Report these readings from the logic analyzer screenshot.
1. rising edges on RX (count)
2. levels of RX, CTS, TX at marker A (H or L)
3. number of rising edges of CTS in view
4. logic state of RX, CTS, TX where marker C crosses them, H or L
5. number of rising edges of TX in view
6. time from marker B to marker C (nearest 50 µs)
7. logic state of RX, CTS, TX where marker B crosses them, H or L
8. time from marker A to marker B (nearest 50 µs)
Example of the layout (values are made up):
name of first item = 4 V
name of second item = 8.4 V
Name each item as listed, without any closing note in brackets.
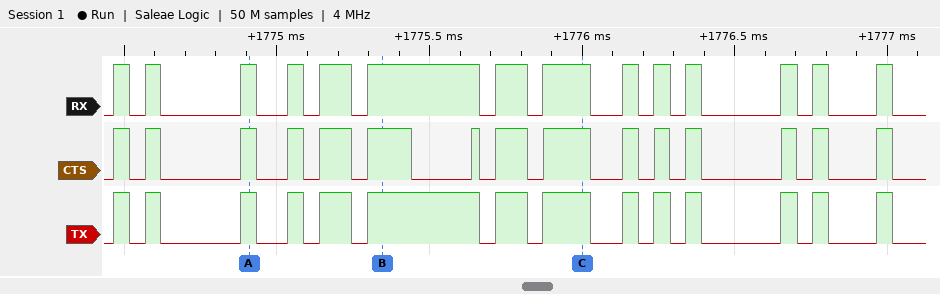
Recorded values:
rising edges on RX = 14
levels of RX, CTS, TX at marker A = RX=H, CTS=H, TX=H
number of rising edges of CTS in view = 15
logic state of RX, CTS, TX where marker C crosses them, H or L = RX=H, CTS=H, TX=H
number of rising edges of TX in view = 14
time from marker B to marker C = 650 µs
logic state of RX, CTS, TX where marker B crosses them, H or L = RX=H, CTS=H, TX=H
time from marker A to marker B = 450 µs
